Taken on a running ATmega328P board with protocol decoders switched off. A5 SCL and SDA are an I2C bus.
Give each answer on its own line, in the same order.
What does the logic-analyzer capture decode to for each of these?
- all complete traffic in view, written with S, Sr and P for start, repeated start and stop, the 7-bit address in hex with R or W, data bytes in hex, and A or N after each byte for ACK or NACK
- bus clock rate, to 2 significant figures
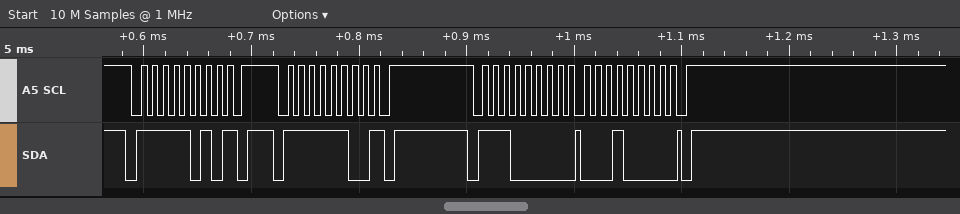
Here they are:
S 7DW N P S 7EW N P S 70W A 10 A P
100 kHz
